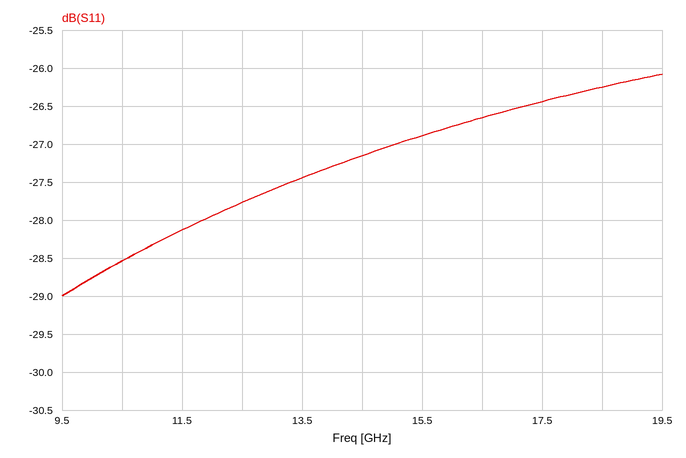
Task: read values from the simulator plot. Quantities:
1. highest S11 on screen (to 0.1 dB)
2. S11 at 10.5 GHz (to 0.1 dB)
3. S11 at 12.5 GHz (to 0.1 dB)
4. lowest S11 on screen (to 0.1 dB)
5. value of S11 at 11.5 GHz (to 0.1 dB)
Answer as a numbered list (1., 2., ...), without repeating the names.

1. -26.1 dB
2. -28.5 dB
3. -27.8 dB
4. -29.0 dB
5. -28.1 dB
